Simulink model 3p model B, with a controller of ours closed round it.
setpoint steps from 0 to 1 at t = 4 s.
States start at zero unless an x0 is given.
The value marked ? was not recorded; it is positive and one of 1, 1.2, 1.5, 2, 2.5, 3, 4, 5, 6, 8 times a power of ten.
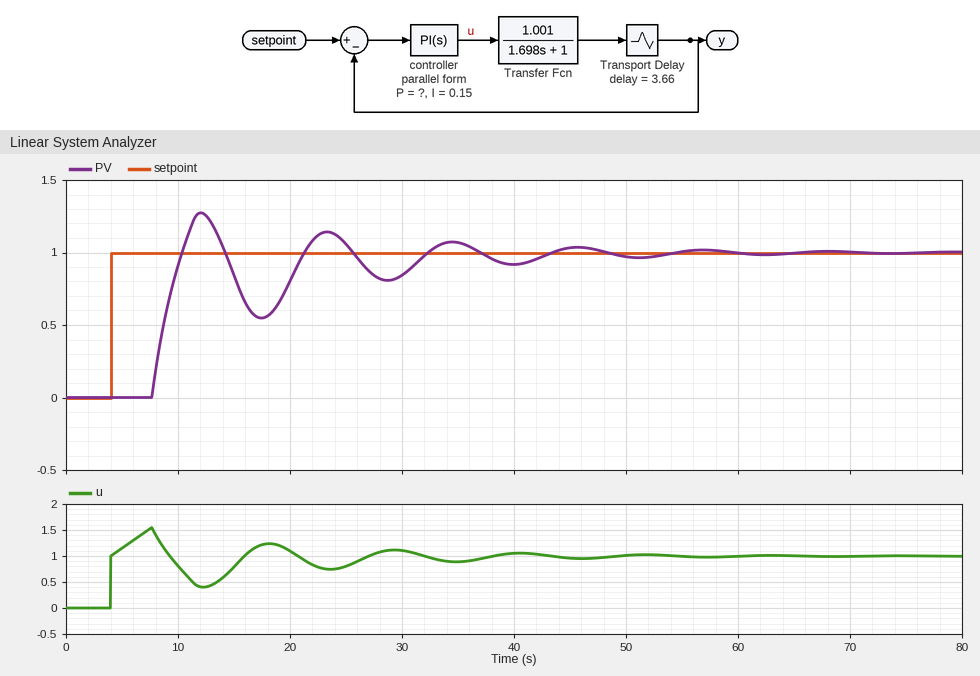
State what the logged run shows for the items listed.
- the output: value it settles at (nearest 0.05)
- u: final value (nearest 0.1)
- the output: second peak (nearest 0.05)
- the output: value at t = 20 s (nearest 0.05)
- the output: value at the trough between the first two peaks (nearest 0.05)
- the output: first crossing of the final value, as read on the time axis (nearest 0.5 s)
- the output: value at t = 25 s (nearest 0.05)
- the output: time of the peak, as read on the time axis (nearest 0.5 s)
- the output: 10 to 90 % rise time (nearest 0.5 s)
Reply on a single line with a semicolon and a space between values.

1.00; 1.0; 1.15; 0.80; 0.55; 10.5 s; 1.05; 12.0 s; 2.0 s
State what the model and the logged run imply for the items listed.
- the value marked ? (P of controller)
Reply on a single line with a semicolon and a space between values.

1
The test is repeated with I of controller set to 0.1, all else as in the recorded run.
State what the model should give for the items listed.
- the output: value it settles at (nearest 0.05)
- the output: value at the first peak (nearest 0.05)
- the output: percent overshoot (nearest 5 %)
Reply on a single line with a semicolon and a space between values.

1.00; 1.15; 15 %
